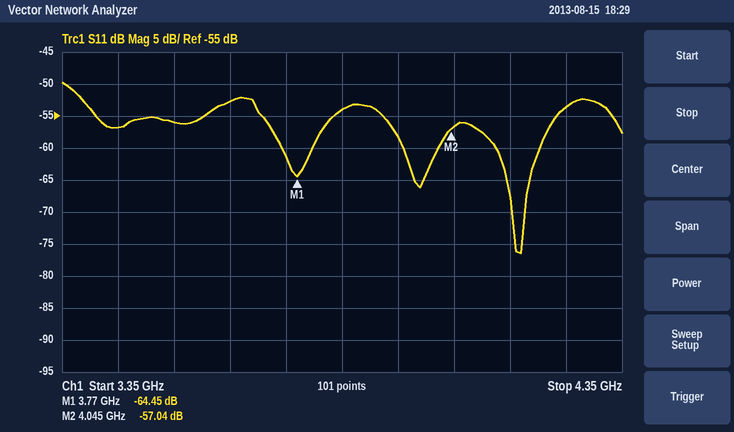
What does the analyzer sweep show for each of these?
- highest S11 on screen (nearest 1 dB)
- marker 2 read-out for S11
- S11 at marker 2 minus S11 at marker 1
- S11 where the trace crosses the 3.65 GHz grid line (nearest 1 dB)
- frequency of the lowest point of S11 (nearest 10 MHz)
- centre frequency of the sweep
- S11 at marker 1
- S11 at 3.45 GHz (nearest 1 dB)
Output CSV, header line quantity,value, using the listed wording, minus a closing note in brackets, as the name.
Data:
quantity,value
highest S11 on screen,-50 dB
marker 2 read-out for S11,-57.04 dB
S11 at marker 2 minus S11 at marker 1,7.41 dB
S11 where the trace crosses the 3.65 GHz grid line,-53 dB
frequency of the lowest point of S11,4.17 GHz
centre frequency of the sweep,3.85 GHz
S11 at marker 1,-64.45 dB
S11 at 3.45 GHz,-57 dB
